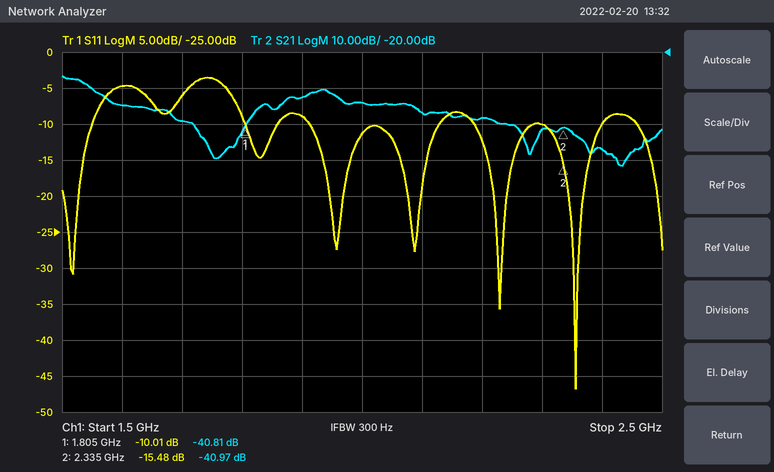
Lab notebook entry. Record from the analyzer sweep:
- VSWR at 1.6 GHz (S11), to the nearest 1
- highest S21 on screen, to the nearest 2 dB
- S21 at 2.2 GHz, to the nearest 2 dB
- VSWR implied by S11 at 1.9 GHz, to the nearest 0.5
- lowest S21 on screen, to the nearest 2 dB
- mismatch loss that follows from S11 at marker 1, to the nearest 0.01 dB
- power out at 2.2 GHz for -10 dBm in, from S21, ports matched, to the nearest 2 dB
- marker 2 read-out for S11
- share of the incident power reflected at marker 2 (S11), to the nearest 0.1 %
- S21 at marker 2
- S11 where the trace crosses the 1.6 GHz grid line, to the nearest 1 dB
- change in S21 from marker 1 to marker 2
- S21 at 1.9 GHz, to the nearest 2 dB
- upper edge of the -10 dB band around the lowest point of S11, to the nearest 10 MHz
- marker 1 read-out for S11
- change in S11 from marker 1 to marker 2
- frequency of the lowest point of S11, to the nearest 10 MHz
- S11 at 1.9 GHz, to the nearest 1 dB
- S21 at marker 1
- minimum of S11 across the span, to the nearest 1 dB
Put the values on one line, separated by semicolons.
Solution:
4; -26 dB; -38 dB; 2.0; -52 dB; 0.46 dB; -48 dBm; -15.48 dB; 2.8 %; -40.97 dB; -5 dB; -0.16 dB; -32 dB; 2.40 GHz; -10.01 dB; -5.47 dB; 2.36 GHz; -9 dB; -40.81 dB; -47 dB
